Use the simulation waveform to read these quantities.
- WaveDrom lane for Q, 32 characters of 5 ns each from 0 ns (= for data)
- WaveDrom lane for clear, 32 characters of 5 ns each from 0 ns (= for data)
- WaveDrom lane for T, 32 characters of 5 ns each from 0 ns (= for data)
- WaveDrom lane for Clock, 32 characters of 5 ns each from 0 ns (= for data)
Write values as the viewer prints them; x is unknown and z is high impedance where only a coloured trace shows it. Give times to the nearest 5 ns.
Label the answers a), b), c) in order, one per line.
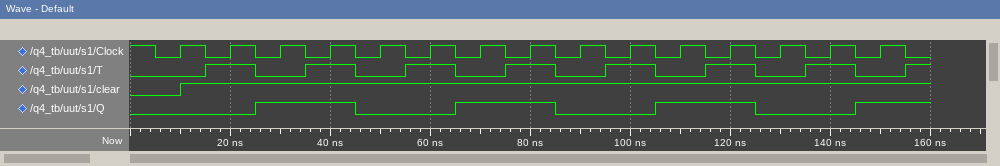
a) {name: 'Q', wave: '0....1...0...1...0...1...0...1..'}
b) {name: 'clear', wave: '0.1.............................'}
c) {name: 'T', wave: '0..1.0.1.0.1.0.1.0.1.0.1.0.1.0.1'}
d) {name: 'Clock', wave: '10101010101010101010101010101010'}
